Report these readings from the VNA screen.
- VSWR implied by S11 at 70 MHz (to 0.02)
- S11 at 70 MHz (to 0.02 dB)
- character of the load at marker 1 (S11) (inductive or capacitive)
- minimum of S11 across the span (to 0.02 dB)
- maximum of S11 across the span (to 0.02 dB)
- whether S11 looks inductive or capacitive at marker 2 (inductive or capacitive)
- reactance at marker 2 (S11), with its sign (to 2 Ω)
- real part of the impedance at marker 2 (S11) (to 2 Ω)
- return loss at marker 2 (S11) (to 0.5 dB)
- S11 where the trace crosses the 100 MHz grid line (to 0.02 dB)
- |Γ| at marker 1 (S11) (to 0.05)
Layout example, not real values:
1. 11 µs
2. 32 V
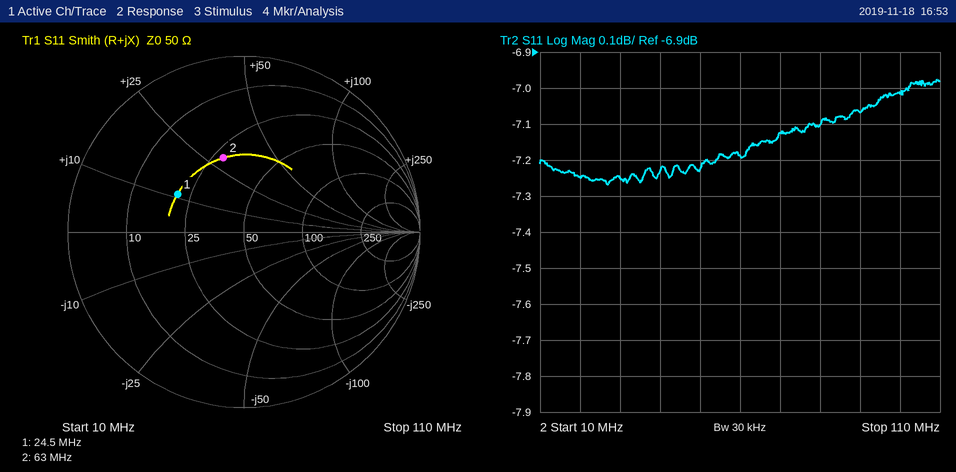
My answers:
1. 2.58
2. -7.12 dB
3. inductive
4. -7.26 dB
5. -6.98 dB
6. inductive
7. +30 Ω
8. 28 Ω
9. 7.0 dB
10. -7.02 dB
11. 0.45
